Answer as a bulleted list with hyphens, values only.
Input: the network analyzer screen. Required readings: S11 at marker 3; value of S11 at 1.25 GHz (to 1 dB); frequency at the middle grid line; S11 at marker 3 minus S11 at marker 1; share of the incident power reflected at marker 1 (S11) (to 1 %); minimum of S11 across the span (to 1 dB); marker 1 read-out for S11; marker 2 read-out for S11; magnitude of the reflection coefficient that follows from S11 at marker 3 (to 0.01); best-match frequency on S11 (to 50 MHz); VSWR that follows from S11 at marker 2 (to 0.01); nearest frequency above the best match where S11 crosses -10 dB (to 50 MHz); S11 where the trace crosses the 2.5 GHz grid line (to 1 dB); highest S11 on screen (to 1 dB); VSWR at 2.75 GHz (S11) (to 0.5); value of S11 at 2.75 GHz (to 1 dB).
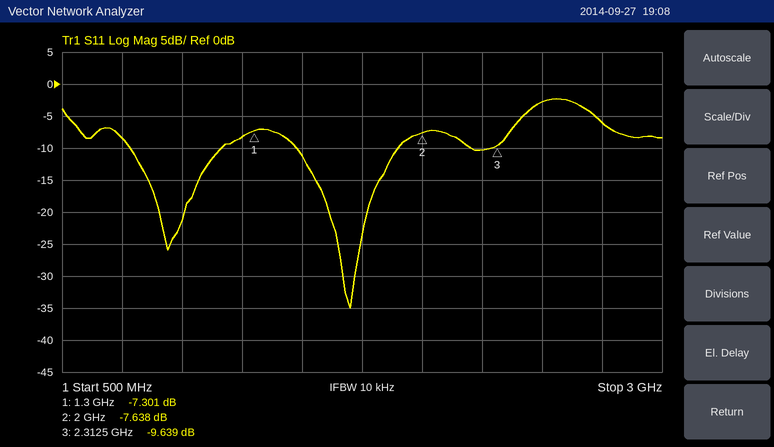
- -9.639 dB
- -8 dB
- 1.75 GHz
- -2.338 dB
- 19 %
- -35 dB
- -7.301 dB
- -7.638 dB
- 0.33
- 1.70 GHz
- 2.42
- 1.90 GHz
- -3 dB
- -2 dB
- 3.0
- -6 dB
